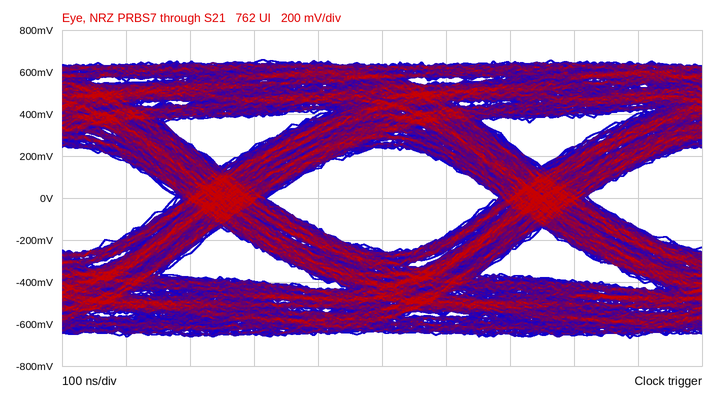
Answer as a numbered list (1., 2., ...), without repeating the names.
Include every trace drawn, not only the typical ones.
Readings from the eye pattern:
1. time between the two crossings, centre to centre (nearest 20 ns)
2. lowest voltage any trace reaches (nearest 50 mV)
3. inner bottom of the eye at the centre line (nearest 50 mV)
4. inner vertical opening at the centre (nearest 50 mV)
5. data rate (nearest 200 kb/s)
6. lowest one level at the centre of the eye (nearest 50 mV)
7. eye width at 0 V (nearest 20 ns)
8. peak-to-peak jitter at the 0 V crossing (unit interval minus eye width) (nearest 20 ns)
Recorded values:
1. 500 ns
2. -650 mV
3. -250 mV
4. 500 mV
5. 2.0 Mb/s
6. 250 mV
7. 360 ns
8. 140 ns
